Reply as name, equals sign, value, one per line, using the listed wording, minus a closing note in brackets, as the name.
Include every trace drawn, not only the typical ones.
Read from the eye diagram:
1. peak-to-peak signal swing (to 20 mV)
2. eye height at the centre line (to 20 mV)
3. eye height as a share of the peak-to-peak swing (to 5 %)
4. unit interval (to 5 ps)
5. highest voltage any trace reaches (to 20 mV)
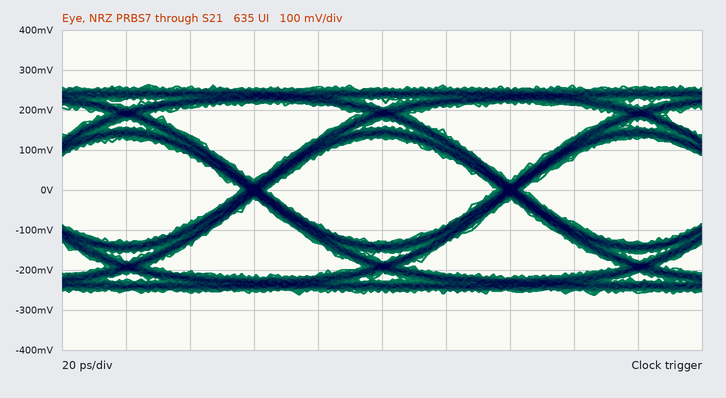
peak-to-peak signal swing = 520 mV
eye height at the centre line = 260 mV
eye height as a share of the peak-to-peak swing = 50 %
unit interval = 80 ps
highest voltage any trace reaches = 260 mV
